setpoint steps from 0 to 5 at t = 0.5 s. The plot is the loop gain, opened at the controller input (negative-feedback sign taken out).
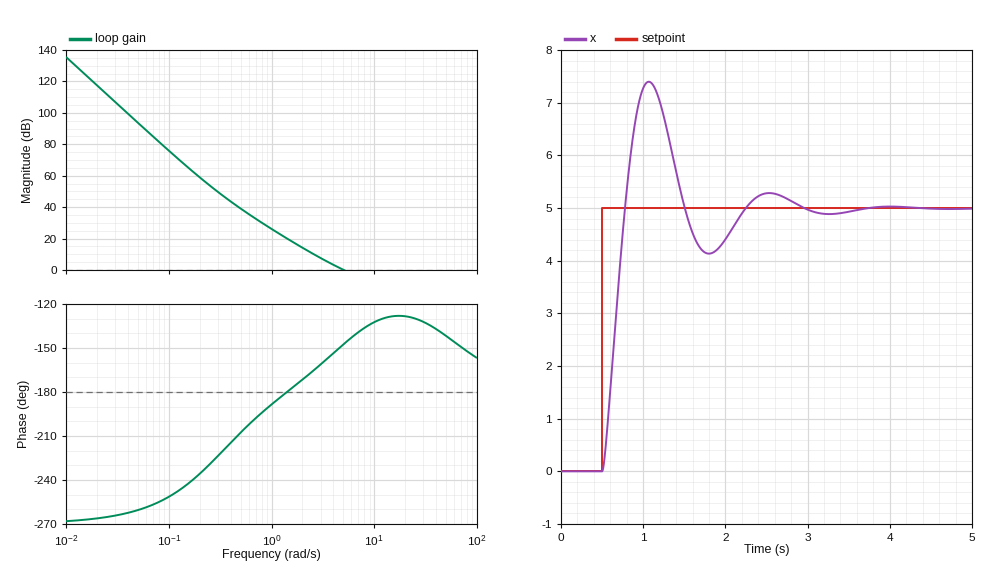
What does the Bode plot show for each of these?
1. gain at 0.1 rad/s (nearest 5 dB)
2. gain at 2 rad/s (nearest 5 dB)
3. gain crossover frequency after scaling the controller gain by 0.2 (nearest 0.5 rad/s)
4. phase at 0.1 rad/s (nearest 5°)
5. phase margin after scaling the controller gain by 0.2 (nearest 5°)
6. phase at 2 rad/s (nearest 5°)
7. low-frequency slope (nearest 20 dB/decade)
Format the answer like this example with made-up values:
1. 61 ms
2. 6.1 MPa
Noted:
1. 75 dB
2. 15 dB
3. 2.0 rad/s
4. -250°
5. 10°
6. -170°
7. -60 dB/decade
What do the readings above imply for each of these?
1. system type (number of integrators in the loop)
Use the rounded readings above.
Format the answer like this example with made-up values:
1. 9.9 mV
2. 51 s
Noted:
1. 3
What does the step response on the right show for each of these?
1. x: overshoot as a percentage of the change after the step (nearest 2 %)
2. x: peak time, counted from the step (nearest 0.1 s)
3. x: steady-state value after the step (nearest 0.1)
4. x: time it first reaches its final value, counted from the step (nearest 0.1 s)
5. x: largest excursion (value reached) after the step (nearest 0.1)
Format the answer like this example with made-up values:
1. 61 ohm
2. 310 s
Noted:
1. 48 %
2. 0.6 s
3. 5.0
4. 0.3 s
5. 7.4
